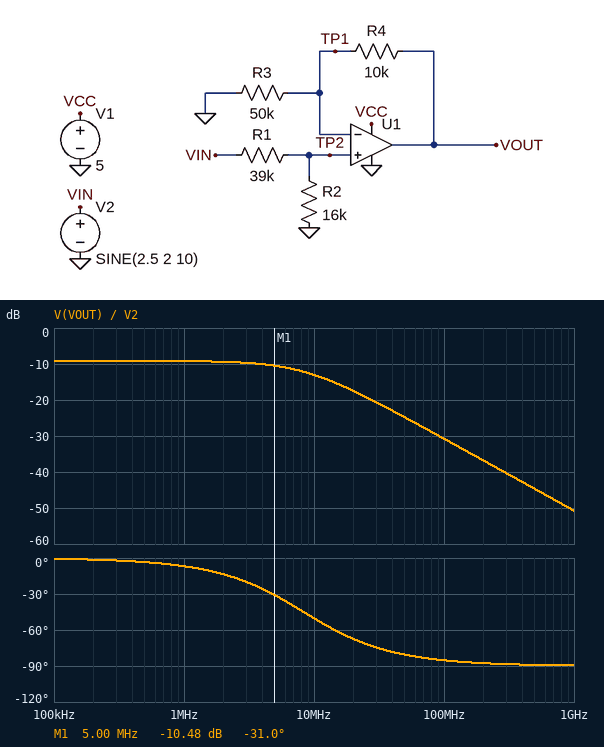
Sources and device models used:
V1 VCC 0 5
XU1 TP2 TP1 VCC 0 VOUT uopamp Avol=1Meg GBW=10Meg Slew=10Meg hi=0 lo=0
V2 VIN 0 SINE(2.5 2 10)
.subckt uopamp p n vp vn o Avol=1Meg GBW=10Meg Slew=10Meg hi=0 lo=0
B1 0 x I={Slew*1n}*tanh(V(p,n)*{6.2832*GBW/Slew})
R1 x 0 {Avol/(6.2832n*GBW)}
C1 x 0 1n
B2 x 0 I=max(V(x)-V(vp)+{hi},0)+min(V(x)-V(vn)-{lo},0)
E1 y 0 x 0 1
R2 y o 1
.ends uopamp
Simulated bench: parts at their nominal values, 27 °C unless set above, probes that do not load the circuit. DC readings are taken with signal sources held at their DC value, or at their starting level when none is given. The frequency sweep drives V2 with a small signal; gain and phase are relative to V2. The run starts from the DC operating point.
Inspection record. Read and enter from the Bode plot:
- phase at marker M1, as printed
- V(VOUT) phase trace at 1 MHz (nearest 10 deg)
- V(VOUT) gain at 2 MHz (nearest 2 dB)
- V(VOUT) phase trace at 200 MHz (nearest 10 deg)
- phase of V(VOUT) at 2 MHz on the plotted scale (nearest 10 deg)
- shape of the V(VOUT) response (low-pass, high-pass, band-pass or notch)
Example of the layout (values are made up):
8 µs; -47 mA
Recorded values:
-31.0 deg; -10 deg; -10 dB; -90 deg; -10 deg; low-pass
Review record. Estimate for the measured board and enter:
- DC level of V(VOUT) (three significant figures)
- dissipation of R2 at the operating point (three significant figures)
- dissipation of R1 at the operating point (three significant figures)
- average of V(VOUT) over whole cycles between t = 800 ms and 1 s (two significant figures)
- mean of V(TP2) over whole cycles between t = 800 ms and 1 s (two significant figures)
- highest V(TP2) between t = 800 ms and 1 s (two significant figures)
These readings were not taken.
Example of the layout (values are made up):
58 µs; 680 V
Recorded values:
873 mV; 33.1 µW; 80.6 µW; 870 mV; 730 mV; 1.3 V
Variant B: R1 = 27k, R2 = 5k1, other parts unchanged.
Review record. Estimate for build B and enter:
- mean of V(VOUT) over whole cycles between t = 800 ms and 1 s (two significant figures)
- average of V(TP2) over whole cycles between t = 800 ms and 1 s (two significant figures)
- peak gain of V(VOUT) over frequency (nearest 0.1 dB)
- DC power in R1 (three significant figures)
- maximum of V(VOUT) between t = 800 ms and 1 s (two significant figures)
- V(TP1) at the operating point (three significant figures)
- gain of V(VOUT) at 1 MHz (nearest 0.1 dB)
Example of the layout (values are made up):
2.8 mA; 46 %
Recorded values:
480 mV; 400 mV; -14.4 dB; 164 µW; 860 mV; 397 mV; -14.5 dB
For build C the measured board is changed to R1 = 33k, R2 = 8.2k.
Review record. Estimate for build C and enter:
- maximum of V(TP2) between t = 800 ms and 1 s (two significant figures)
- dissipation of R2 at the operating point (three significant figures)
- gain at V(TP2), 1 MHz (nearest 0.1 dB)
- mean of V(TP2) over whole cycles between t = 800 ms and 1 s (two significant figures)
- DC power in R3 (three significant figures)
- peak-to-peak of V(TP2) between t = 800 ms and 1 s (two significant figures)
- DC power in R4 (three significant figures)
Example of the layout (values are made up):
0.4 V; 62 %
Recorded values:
900 mV; 30.2 µW; -14.0 dB; 500 mV; 4.95 µW; 800 mV; 990 nW
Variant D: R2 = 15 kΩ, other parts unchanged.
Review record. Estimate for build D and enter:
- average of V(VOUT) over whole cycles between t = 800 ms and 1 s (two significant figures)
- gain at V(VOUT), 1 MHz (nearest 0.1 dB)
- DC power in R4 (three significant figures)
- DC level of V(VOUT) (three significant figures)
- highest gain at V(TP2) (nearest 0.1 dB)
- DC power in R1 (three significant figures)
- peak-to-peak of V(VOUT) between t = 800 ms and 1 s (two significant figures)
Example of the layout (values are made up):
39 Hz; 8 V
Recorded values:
830 mV; -9.6 dB; 1.93 µW; 833 mV; -11.1 dB; 83.6 µW; 1.3 V
